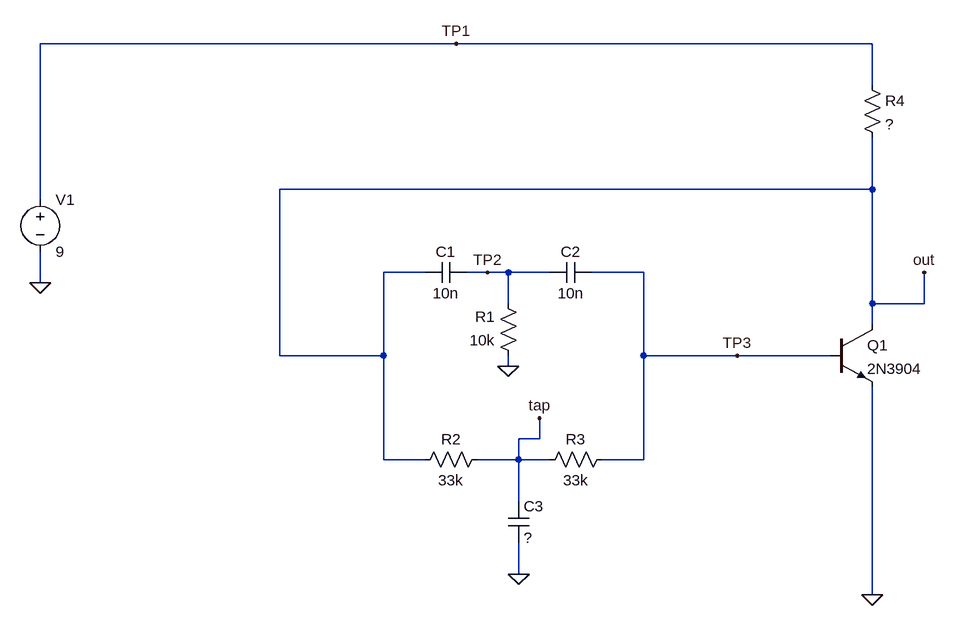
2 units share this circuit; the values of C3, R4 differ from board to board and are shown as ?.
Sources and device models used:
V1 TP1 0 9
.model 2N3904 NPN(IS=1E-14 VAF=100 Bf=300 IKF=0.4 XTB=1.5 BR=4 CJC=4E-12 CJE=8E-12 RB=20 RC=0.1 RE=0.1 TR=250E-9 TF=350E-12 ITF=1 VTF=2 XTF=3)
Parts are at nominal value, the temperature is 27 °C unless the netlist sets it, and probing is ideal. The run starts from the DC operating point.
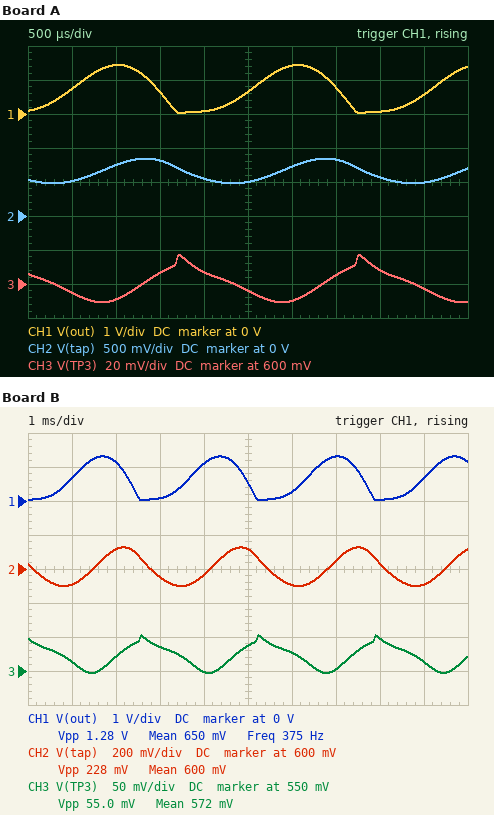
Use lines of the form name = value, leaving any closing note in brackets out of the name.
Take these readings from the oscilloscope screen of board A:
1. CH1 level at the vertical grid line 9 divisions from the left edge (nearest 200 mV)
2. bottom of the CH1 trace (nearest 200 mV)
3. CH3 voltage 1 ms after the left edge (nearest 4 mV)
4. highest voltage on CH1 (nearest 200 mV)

CH1 level at the vertical grid line 9 divisions from the left edge = 600 mV
bottom of the CH1 trace = 0 V
CH3 voltage 1 ms after the left edge = 592 mV
highest voltage on CH1 = 1.4 V
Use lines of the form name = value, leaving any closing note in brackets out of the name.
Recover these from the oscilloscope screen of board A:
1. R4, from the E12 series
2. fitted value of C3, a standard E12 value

R4, from the E12 series = 68 kΩ
fitted value of C3, a standard E12 value = 33 nF
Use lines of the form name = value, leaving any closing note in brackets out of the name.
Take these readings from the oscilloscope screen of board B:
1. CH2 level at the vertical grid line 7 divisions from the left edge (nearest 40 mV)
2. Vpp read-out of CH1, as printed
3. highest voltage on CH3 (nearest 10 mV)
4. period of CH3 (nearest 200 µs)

CH2 level at the vertical grid line 7 divisions from the left edge = 640 mV
Vpp read-out of CH1, as printed = 1.28 V
highest voltage on CH3 = 600 mV
period of CH3 = 2.6 ms
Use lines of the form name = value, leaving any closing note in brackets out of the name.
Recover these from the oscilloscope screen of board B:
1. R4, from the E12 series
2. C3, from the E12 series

R4, from the E12 series = 180 kΩ
C3, from the E12 series = 68 nF
